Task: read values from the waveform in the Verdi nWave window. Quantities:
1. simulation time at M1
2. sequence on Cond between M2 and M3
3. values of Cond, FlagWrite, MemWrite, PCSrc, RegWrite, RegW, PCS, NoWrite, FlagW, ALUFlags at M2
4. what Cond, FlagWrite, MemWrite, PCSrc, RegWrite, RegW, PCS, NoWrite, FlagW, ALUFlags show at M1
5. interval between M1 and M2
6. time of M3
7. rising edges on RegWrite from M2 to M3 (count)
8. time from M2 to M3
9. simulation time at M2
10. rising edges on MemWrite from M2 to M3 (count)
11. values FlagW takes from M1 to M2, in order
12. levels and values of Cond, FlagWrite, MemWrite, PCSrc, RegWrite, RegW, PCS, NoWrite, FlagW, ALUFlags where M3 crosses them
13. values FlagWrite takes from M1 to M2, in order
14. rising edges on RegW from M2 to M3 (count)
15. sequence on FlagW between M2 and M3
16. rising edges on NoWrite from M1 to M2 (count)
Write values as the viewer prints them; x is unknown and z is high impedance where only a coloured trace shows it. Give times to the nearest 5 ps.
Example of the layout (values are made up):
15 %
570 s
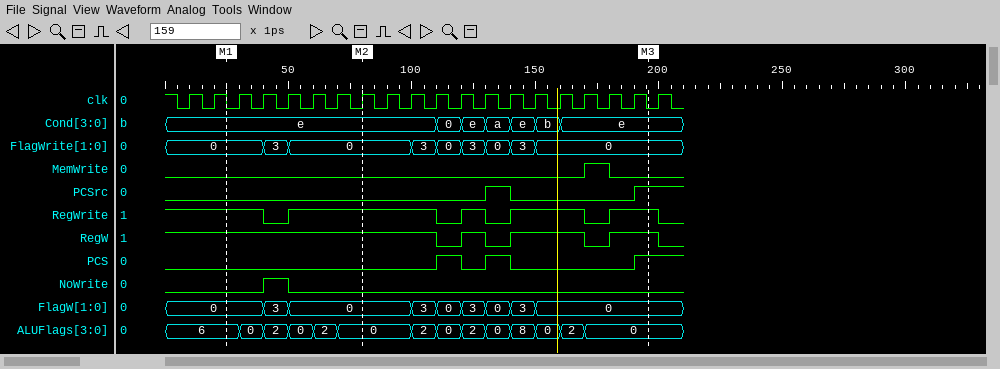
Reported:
25 ps
e, 0, e, a, e, b, e
Cond=e, FlagWrite=0, MemWrite=0, PCSrc=0, RegWrite=1, RegW=1, PCS=0, NoWrite=0, FlagW=0, ALUFlags=0
Cond=e, FlagWrite=0, MemWrite=0, PCSrc=0, RegWrite=1, RegW=1, PCS=0, NoWrite=0, FlagW=0, ALUFlags=6
55 ps
195 ps
3
115 ps
80 ps
1
0, 3, 0
Cond=e, FlagWrite=0, MemWrite=0, PCSrc=1, RegWrite=1, RegW=1, PCS=1, NoWrite=0, FlagW=0, ALUFlags=0
0, 3, 0
3
0, 3, 0, 3, 0, 3, 0
1
